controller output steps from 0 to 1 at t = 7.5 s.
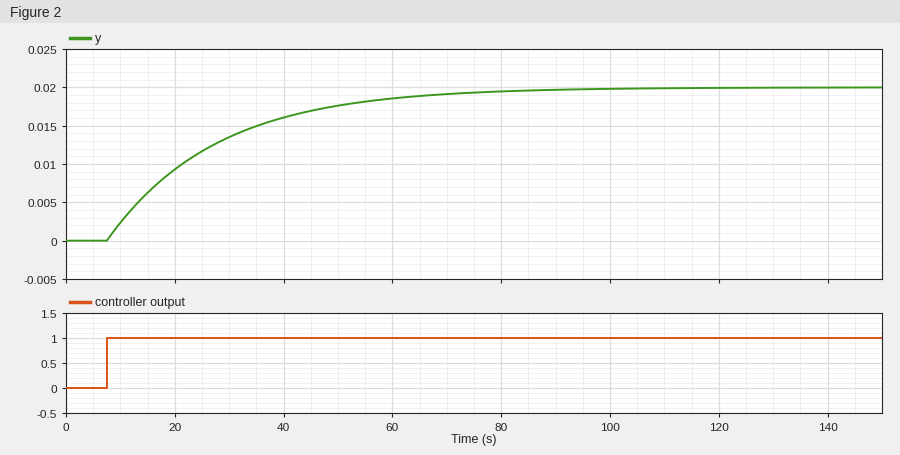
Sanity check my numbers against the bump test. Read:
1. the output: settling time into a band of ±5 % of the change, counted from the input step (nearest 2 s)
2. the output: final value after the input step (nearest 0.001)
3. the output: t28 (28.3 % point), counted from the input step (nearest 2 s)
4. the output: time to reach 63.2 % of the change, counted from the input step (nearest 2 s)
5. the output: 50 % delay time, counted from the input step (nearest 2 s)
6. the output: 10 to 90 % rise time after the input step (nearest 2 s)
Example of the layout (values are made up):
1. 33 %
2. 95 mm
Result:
1. 60 s
2. 0.020
3. 6 s
4. 20 s
5. 14 s
6. 44 s
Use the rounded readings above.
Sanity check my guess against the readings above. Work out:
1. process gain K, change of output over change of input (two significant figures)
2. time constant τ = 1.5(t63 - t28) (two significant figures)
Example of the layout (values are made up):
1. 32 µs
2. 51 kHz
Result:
1. 0.020
2. 21 s
